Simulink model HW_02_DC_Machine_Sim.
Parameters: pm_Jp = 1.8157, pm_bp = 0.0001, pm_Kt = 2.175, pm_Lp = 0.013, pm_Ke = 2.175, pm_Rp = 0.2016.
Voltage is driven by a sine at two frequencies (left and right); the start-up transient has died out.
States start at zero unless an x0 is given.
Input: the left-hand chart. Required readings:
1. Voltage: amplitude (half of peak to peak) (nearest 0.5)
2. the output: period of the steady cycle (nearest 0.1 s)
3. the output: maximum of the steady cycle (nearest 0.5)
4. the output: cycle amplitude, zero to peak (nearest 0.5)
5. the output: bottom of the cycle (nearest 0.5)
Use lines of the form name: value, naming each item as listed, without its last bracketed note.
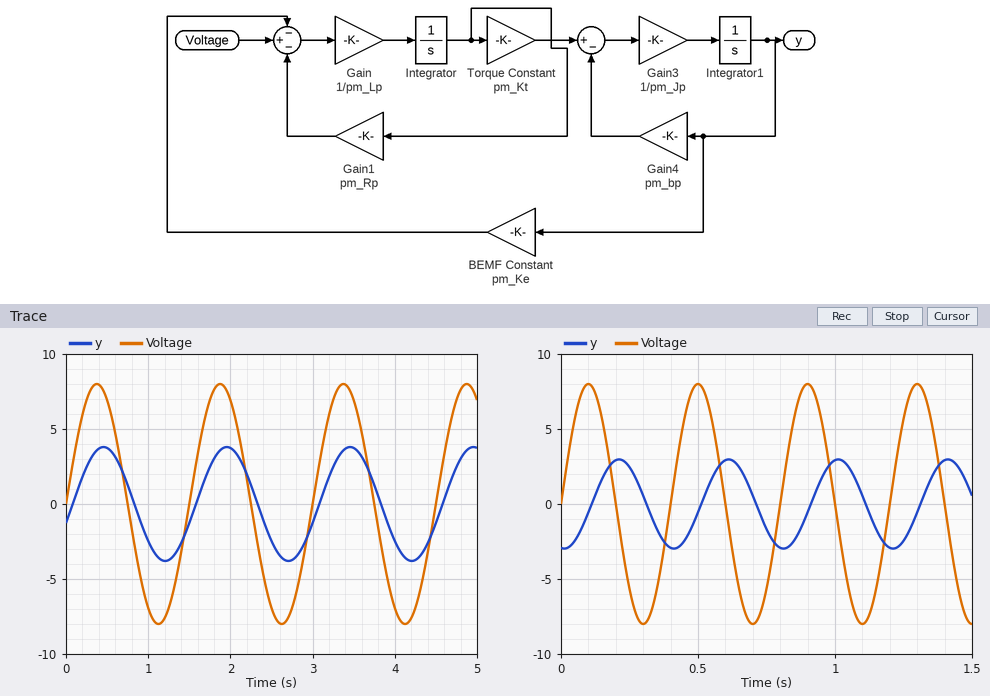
Voltage: amplitude (half of peak to peak): 8.0
the output: period of the steady cycle: 1.5 s
the output: maximum of the steady cycle: 4.0
the output: cycle amplitude, zero to peak: 4.0
the output: bottom of the cycle: -4.0
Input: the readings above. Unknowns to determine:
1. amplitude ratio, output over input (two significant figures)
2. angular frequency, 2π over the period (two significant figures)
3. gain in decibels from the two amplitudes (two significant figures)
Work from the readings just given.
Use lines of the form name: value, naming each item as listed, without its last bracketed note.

amplitude ratio, output over input: 0.50
angular frequency, 2π over the period: 4.2 rad/s
gain in decibels from the two amplitudes: -6.0 dB
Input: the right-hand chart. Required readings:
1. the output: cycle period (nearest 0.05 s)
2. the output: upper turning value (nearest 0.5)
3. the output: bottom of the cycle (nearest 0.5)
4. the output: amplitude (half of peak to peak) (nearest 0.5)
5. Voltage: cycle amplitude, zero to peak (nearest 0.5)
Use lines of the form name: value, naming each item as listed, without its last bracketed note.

the output: cycle period: 0.40 s
the output: upper turning value: 3.0
the output: bottom of the cycle: -3.0
the output: amplitude (half of peak to peak): 3.0
Voltage: cycle amplitude, zero to peak: 8.0
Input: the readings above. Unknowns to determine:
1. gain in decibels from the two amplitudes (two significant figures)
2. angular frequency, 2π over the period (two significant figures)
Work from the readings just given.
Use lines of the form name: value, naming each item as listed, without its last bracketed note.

gain in decibels from the two amplitudes: -8.5 dB
angular frequency, 2π over the period: 16 rad/s
